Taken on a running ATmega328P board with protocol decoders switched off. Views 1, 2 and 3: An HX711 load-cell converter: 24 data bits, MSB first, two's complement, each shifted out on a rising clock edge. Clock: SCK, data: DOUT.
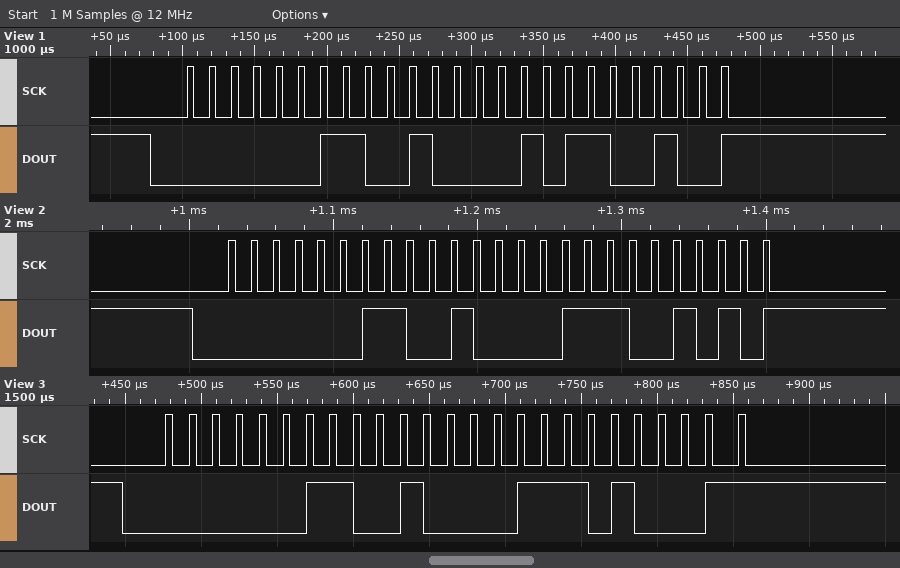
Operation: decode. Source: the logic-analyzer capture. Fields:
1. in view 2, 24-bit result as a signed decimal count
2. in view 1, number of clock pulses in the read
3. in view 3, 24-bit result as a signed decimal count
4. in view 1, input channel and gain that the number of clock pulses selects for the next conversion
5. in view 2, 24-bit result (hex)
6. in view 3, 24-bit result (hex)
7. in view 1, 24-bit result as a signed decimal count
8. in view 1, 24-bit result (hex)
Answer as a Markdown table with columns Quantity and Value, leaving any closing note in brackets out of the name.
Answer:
| Quantity | Value |
|---|---|
| in view 2, 24-bit result as a signed decimal count | 205258 |
| in view 1, number of clock pulses in the read | 25 |
| in view 3, 24-bit result as a signed decimal count | 205265 |
| in view 1, input channel and gain that the number of clock pulses selects for the next conversion | channel A, gain 128 |
| in view 2, 24-bit result | 0x0321CA |
| in view 3, 24-bit result | 0x0321D1 |
| in view 1, 24-bit result as a signed decimal count | 205156 |
| in view 1, 24-bit result | 0x032164 |
